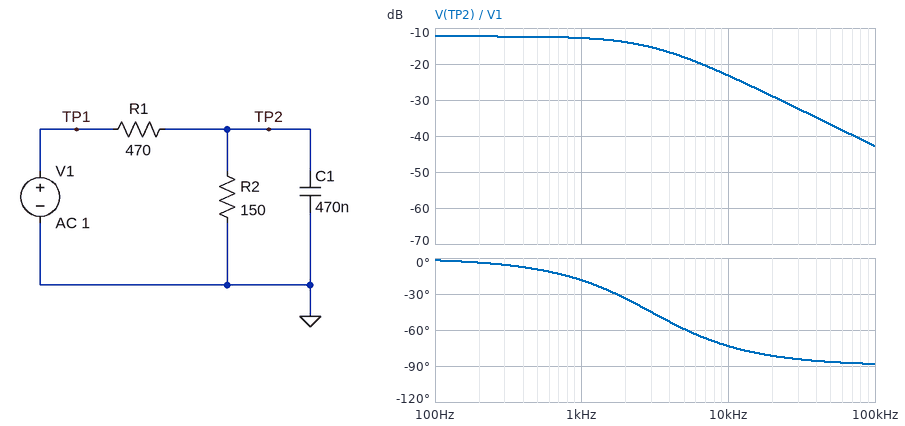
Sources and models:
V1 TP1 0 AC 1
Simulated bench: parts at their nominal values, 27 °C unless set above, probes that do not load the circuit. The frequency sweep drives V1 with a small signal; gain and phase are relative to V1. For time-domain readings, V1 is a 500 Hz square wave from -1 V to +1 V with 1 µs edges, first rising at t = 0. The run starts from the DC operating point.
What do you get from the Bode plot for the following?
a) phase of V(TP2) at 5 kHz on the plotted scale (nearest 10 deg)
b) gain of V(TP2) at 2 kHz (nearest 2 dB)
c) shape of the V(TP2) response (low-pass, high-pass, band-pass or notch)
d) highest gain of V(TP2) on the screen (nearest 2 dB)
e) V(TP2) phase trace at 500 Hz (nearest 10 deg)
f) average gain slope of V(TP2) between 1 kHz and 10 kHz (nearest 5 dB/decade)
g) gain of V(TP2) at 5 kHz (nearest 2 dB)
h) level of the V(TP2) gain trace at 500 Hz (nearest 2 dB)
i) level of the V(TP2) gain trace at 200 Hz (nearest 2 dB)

-60 deg
-14 dB
low-pass
-12 dB
-10 deg
-10 dB/decade
-18 dB
-12 dB
-12 dB
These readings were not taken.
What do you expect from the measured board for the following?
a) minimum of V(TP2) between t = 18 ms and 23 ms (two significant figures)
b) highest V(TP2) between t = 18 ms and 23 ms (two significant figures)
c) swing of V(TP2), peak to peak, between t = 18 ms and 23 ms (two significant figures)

-240 mV
240 mV
480 mV
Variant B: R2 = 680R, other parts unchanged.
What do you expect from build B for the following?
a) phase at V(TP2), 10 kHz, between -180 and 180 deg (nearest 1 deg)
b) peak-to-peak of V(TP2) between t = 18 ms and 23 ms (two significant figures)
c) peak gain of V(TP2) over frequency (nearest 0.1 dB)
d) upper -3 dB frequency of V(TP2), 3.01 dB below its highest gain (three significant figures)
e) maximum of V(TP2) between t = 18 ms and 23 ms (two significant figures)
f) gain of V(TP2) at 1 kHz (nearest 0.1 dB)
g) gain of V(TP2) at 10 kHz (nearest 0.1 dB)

-83 deg
1.2 V
-4.6 dB
1.22 kHz
590 mV
-6.8 dB
-22.9 dB
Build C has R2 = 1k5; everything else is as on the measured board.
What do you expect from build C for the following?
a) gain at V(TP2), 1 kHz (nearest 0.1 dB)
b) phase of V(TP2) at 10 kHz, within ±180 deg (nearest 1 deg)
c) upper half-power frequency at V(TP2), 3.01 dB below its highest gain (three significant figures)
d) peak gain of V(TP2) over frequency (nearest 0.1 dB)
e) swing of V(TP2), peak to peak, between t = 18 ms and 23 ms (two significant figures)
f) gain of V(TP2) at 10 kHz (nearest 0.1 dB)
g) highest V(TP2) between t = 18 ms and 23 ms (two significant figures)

-5.6 dB
-85 deg
946 Hz
-2.4 dB
1.5 V
-22.9 dB
760 mV
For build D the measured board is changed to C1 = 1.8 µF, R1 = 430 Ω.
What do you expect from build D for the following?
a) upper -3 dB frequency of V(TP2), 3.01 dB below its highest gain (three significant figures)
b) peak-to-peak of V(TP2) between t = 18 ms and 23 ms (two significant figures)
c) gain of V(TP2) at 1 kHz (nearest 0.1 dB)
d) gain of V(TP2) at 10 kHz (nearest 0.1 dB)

795 Hz
510 mV
-15.9 dB
-33.8 dB
